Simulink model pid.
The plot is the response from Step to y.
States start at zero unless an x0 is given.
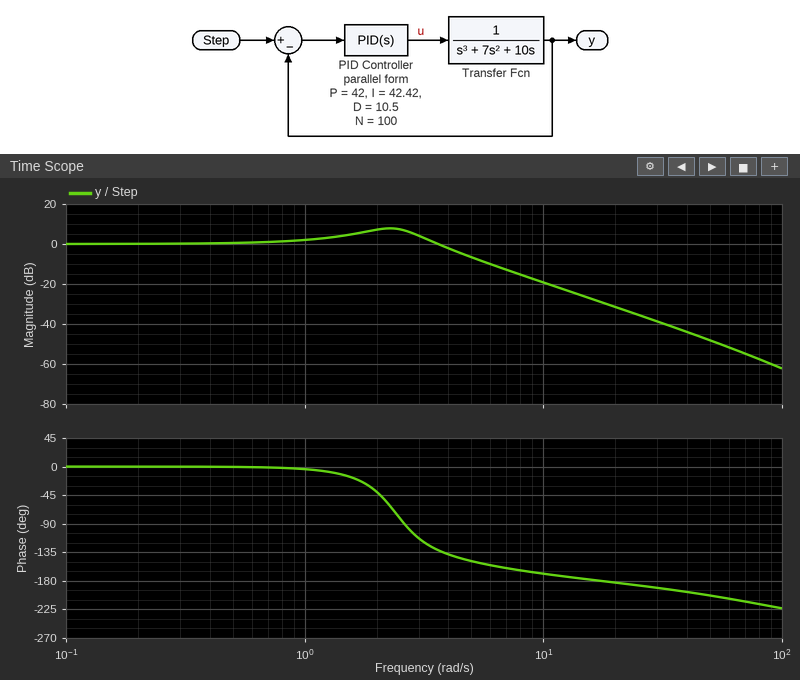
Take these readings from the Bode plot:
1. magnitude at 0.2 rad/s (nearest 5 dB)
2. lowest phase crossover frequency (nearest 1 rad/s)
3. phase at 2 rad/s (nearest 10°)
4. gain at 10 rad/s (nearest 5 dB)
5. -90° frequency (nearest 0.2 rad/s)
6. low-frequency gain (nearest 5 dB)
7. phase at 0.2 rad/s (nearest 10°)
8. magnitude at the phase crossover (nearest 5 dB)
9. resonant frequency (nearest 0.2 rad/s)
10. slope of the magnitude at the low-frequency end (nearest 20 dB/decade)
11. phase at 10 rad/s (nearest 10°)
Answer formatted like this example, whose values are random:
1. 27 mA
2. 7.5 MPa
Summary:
1. 0 dB
2. 17 rad/s
3. -40°
4. -20 dB
5. 2.6 rad/s
6. 0 dB
7. 0°
8. -30 dB
9. 2.2 rad/s
10. 0 dB/decade
11. -170°
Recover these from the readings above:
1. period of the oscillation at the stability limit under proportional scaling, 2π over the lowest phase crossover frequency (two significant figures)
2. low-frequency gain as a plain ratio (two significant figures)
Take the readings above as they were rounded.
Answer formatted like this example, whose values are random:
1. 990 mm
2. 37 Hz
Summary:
1. 0.37 s
2. 1.0
